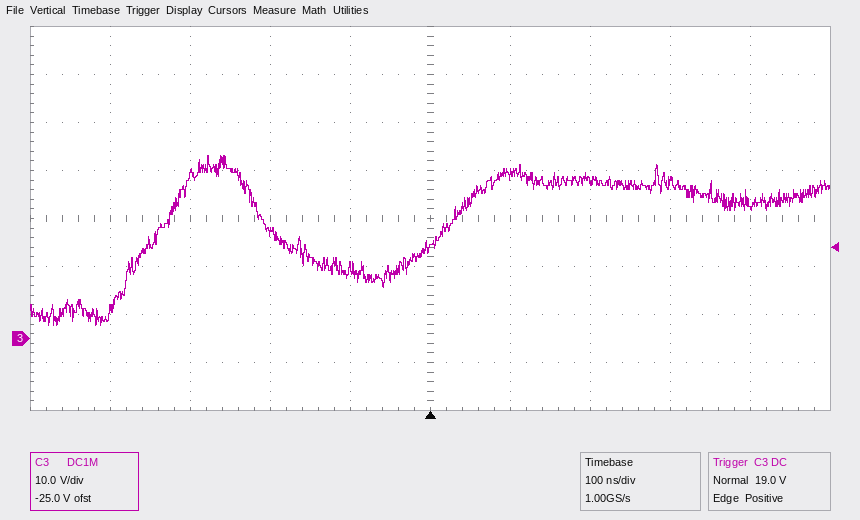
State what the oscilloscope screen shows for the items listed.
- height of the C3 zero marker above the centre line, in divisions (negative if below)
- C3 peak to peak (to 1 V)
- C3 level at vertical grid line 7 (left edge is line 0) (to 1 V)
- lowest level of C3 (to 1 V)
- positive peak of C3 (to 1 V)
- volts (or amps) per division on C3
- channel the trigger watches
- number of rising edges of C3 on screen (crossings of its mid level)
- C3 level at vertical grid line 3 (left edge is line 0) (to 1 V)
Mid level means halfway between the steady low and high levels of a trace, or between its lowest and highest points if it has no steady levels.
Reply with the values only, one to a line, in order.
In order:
-2.5 div
35 V
33 V
3 V
38 V
10 V
C3
2
22 V
